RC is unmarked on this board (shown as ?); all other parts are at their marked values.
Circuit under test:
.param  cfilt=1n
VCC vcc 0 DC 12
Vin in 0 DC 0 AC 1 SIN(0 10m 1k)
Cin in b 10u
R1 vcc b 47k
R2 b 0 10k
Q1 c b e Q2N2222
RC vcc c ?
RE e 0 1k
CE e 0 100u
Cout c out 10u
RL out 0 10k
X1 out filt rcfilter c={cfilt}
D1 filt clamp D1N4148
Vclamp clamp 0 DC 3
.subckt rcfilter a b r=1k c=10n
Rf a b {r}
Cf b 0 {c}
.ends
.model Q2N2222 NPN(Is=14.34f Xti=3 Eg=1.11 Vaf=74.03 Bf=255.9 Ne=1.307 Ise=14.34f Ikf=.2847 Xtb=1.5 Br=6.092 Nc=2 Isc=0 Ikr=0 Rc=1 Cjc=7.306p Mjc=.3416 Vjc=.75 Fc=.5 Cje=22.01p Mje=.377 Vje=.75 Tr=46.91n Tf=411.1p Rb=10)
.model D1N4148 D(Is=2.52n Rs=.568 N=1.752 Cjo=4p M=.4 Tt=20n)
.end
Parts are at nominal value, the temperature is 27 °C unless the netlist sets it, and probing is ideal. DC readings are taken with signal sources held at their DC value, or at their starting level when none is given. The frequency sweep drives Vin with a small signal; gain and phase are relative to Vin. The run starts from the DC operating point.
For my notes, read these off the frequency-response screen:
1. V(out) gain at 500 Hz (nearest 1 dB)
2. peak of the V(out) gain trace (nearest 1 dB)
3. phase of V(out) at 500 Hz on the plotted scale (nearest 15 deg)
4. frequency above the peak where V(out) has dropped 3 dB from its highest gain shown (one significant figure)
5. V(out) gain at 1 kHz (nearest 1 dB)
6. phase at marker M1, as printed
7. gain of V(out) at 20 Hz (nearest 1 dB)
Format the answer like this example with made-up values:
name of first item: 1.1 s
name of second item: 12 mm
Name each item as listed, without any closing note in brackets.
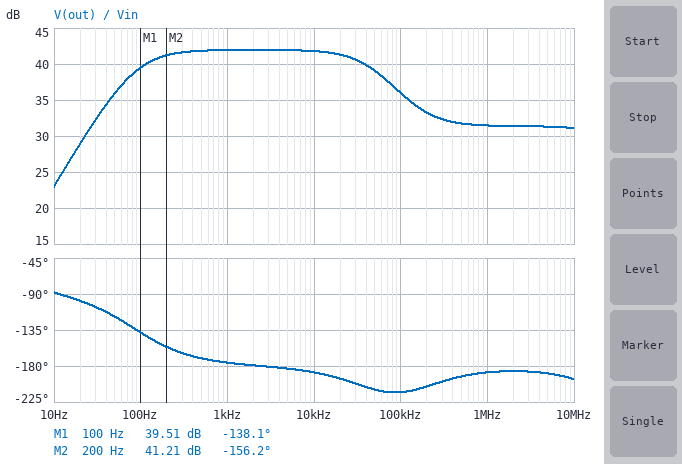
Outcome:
V(out) gain at 500 Hz: 42 dB
peak of the V(out) gain trace: 42 dB
phase of V(out) at 500 Hz on the plotted scale: -165 deg
frequency above the peak where V(out) has dropped 3 dB from its highest gain shown: 50 kHz
V(out) gain at 1 kHz: 42 dB
phase at marker M1, as printed: -138.1 deg
gain of V(out) at 20 Hz: 29 dB
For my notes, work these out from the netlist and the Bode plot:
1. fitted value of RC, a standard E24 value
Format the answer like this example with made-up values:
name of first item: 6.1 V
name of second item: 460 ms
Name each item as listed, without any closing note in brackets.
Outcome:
fitted value of RC, a standard E24 value: 3.3 kΩ
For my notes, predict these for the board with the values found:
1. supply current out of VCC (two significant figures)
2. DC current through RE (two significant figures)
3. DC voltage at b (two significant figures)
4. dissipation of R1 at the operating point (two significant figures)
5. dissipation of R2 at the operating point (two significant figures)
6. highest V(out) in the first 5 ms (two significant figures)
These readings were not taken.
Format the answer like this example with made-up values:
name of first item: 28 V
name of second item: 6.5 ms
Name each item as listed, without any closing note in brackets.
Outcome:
supply current out of VCC: 1.6 mA
DC current through RE: 1.4 mA
DC voltage at b: 2.0 V
dissipation of R1 at the operating point: 2.1 mW
dissipation of R2 at the operating point: 410 µW
highest V(out) in the first 5 ms: 1.1 V
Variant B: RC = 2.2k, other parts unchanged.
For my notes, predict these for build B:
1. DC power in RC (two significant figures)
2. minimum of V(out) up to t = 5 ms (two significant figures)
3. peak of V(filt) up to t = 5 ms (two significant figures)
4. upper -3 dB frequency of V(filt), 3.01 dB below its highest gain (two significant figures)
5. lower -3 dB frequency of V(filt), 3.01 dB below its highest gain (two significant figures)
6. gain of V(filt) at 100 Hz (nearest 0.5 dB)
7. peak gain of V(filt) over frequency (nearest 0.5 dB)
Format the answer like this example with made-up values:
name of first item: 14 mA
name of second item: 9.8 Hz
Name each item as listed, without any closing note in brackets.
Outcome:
DC power in RC: 4.2 mW
minimum of V(out) up to t = 5 ms: -990 mV
peak of V(filt) up to t = 5 ms: 830 mV
upper -3 dB frequency of V(filt), 3.01 dB below its highest gain: 58 kHz
lower -3 dB frequency of V(filt), 3.01 dB below its highest gain: 88 Hz
gain of V(filt) at 100 Hz: 37.0 dB
peak gain of V(filt) over frequency: 39.5 dB
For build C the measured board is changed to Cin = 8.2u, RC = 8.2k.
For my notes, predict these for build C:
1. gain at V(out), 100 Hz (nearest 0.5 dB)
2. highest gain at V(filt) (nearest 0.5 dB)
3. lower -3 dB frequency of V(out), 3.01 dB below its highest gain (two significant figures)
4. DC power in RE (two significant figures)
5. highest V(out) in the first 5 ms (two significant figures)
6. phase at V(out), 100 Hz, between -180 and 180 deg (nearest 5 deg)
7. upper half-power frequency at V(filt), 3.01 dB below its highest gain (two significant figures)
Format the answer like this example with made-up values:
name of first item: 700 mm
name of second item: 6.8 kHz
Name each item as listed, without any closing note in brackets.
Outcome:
gain at V(out), 100 Hz: 20.5 dB
highest gain at V(filt): 25.5 dB
lower -3 dB frequency of V(out), 3.01 dB below its highest gain: 150 Hz
DC power in RE: 1.7 mW
highest V(out) in the first 5 ms: 1.9 V
phase at V(out), 100 Hz, between -180 and 180 deg: -125 deg
upper half-power frequency at V(filt), 3.01 dB below its highest gain: 110 kHz
